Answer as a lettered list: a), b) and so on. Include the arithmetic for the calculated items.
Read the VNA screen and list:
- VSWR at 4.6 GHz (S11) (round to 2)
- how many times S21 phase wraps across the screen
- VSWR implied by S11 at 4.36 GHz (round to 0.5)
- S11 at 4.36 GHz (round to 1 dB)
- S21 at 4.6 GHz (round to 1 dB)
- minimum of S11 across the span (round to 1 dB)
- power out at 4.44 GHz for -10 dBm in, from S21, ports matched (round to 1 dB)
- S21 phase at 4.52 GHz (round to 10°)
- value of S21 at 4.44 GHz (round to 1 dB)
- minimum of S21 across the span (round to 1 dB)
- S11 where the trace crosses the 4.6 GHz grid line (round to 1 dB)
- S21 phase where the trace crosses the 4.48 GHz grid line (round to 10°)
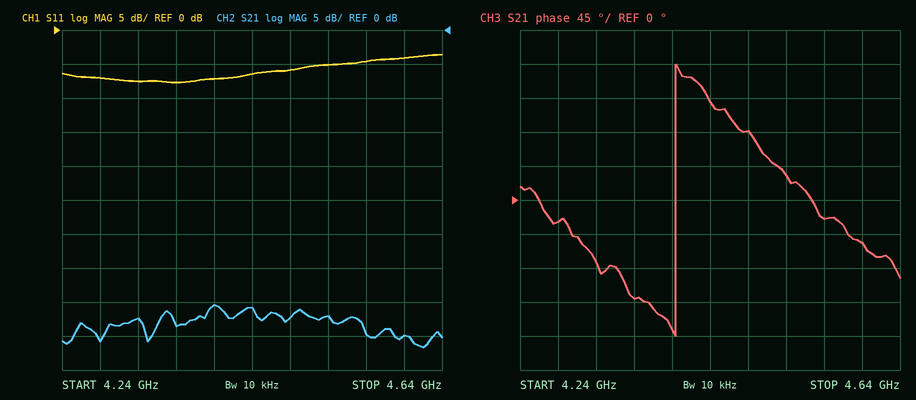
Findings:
a) |Γ| = 10^(-4/20) = 0.6310; VSWR = (1 + 0.6310)/(1 − 0.6310) ≈ 4
b) 1
c) |Γ| = 10^(-8/20) = 0.3981; VSWR = (1 + 0.3981)/(1 − 0.3981) ≈ 2.32, so 2.5 to the nearest 0.5
d) -8 dB
e) -45 dB
f) -8 dB
g) -10 dBm + (-41 dB) = -51 dBm
h) 30°
i) -41 dB
j) -47 dB
k) -4 dB
l) 90°
